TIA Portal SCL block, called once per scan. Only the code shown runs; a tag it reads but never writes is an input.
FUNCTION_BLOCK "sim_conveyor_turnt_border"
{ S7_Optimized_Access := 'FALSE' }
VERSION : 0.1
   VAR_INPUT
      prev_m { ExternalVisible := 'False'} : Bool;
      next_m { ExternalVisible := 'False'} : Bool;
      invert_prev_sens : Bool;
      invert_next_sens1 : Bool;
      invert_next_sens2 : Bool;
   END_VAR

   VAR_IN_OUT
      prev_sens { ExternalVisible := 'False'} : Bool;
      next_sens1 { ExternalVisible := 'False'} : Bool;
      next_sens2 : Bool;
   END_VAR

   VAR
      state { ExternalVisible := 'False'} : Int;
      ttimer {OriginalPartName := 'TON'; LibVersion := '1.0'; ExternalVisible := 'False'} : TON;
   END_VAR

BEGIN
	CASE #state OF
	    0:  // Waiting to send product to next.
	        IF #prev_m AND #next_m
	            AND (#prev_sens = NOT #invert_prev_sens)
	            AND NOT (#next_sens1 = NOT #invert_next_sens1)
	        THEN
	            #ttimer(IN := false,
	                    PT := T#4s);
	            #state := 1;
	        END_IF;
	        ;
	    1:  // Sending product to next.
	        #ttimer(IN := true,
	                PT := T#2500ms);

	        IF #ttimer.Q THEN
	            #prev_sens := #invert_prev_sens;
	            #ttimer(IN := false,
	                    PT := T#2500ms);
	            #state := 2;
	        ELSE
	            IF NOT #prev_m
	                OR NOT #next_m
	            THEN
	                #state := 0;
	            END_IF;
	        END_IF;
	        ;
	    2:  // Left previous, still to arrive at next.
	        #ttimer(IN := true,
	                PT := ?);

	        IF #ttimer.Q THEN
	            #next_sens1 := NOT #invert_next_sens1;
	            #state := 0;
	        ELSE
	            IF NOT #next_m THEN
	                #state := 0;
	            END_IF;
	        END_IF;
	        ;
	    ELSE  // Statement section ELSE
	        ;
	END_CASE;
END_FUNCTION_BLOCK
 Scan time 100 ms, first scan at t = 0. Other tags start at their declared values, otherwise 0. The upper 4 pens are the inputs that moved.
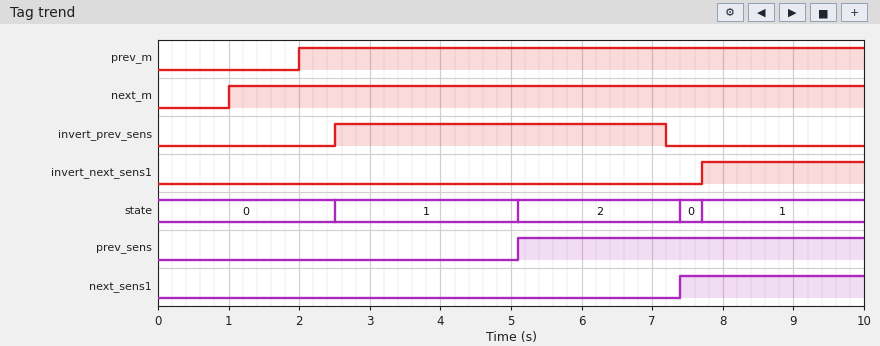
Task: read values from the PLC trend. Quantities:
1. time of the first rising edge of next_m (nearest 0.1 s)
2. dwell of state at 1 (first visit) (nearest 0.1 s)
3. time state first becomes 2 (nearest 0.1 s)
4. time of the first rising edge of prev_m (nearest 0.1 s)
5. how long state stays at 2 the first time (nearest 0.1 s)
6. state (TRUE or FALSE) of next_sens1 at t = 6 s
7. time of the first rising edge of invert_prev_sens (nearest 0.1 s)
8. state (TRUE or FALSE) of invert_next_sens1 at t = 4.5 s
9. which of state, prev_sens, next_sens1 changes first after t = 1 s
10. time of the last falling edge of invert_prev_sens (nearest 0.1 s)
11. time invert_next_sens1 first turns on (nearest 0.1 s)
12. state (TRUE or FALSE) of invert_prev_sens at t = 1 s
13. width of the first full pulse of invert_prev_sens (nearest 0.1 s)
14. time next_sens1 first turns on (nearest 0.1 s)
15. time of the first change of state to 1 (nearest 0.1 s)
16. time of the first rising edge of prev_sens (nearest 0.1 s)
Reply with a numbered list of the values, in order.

1. 1.0 s
2. 2.6 s
3. 5.1 s
4. 2.0 s
5. 2.3 s
6. FALSE
7. 2.5 s
8. FALSE
9. state
10. 7.2 s
11. 7.7 s
12. FALSE
13. 4.7 s
14. 7.4 s
15. 2.5 s
16. 5.1 s
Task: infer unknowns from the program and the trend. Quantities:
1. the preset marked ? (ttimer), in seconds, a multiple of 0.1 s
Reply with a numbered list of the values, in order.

1. 2.2 s
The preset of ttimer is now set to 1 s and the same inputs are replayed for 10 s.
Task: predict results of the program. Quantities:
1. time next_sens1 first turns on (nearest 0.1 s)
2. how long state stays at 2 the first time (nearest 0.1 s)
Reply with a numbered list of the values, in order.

1. 6.2 s
2. 1.1 s
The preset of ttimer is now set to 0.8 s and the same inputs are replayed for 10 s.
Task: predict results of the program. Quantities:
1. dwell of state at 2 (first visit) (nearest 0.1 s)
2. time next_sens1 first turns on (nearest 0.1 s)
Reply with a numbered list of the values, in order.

1. 0.9 s
2. 6.0 s
